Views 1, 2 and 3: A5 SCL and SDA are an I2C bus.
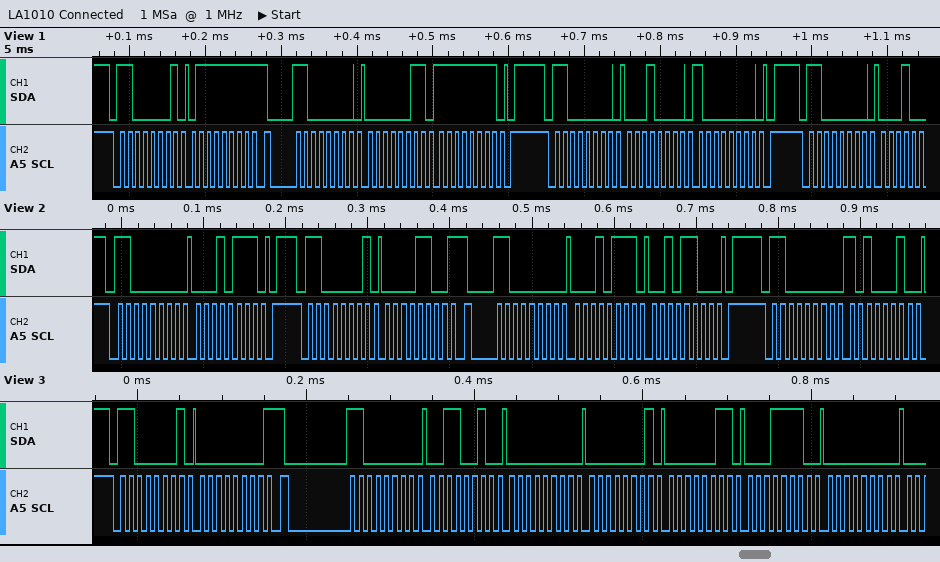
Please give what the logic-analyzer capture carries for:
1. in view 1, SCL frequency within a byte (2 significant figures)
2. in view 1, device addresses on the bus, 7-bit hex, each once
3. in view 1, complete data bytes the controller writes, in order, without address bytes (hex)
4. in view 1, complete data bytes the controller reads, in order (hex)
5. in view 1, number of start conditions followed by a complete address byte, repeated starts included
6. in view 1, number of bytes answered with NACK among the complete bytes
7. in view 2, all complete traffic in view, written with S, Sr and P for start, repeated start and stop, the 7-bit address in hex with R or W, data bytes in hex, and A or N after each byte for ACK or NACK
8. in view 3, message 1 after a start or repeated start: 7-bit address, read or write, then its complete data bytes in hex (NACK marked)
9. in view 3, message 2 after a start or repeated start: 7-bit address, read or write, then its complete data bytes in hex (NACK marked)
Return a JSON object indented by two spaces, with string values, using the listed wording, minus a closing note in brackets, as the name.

{
  "in view 1, SCL frequency within a byte": "100 kHz",
  "in view 1, device addresses on the bus, 7-bit hex, each once": "0x60",
  "in view 1, complete data bytes the controller writes, in order, without address bytes": "03 FF 10 80",
  "in view 1, complete data bytes the controller reads, in order": "7F",
  "in view 1, number of start conditions followed by a complete address byte, repeated starts included": "4",
  "in view 1, number of bytes answered with NACK among the complete bytes": "1",
  "in view 2, all complete traffic in view, written with S, Sr and P for start, repeated start and stop, the 7-bit address in hex with R or W, data bytes in hex, and A or N after each byte for ACK or NACK": "S 60W A 17 A P S 60R A 0C N Sr 60W A 17 A 2C A P S 60W A A2 A",
  "in view 3, message 1 after a start or repeated start: 7-bit address, read or write, then its complete data bytes in hex": "0x60 read: 00 NACK",
  "in view 3, message 2 after a start or repeated start: 7-bit address, read or write, then its complete data bytes in hex": "0x60 write: 32 00 01 03 1E 00"
}
